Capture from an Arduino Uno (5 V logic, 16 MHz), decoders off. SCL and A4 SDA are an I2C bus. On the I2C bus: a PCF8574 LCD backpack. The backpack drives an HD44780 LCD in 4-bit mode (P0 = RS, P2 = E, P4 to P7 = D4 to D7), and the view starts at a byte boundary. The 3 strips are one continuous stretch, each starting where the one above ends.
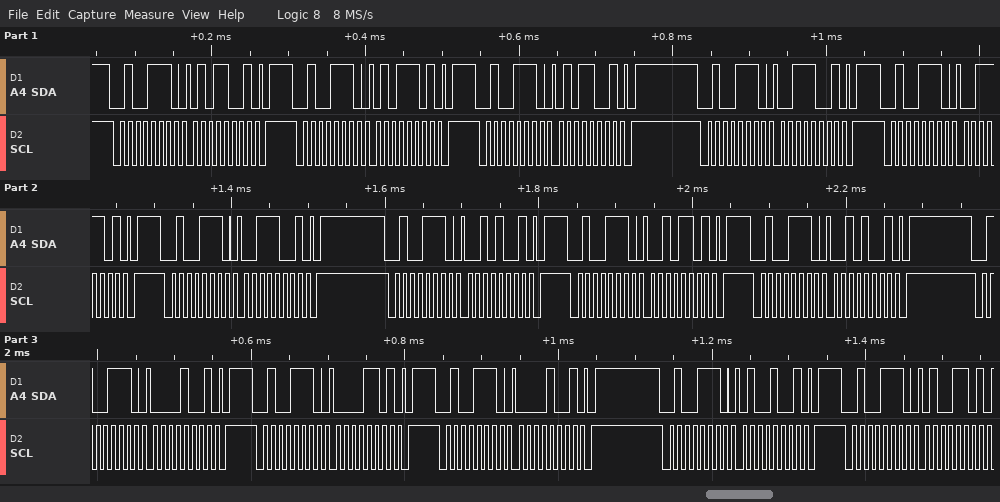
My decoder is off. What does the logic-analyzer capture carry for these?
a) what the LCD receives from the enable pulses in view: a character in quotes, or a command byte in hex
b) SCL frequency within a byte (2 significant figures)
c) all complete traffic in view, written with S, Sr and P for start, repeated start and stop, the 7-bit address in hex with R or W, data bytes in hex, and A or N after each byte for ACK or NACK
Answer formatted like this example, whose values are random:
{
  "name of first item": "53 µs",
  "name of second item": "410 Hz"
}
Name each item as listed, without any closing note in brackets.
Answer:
{
  "what the LCD receives from the enable pulses in view: a character in quotes, or a command byte in hex": "'S' ' '",
  "SCL frequency within a byte": "100 kHz",
  "all complete traffic in view, written with S, Sr and P for start, repeated start and stop, the 7-bit address in hex with R or W, data bytes in hex, and A or N after each byte for ACK or NACK": "S 27W A 59 A P S 27W A 5D A P S 27W A 59 A P S 27W A 39 A P S 27W A 3D A P S 27W A 39 A P S 27W A 29 A P S 27W A 2D A P S 27W A 29 A P S 27W A 09 A P S 27W A 0D A P S 27W A 09 A P S 27W A 49 A P S 27W A 4D A"
}
